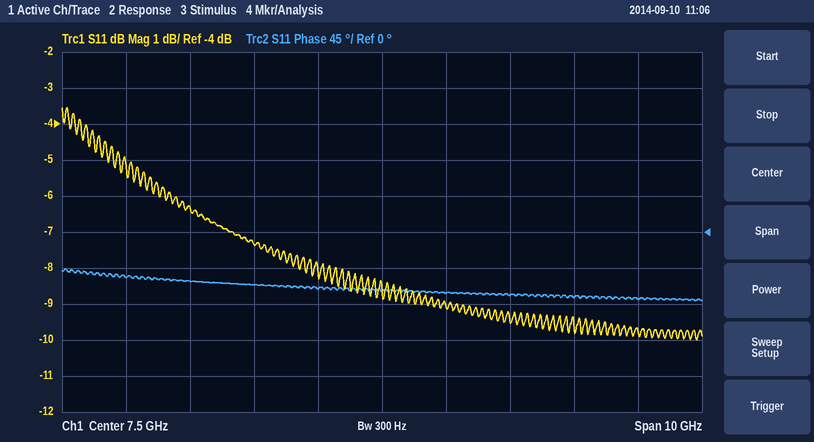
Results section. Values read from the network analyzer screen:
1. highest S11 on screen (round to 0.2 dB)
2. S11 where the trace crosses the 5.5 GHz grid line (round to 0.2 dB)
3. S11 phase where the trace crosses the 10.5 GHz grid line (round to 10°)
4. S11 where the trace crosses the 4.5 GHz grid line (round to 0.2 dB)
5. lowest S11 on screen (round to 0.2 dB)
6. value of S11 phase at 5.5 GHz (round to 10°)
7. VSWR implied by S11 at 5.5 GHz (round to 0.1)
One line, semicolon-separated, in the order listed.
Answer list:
-3.6 dB; -7.4 dB; -80°; -6.4 dB; -10.0 dB; -70°; 2.5
